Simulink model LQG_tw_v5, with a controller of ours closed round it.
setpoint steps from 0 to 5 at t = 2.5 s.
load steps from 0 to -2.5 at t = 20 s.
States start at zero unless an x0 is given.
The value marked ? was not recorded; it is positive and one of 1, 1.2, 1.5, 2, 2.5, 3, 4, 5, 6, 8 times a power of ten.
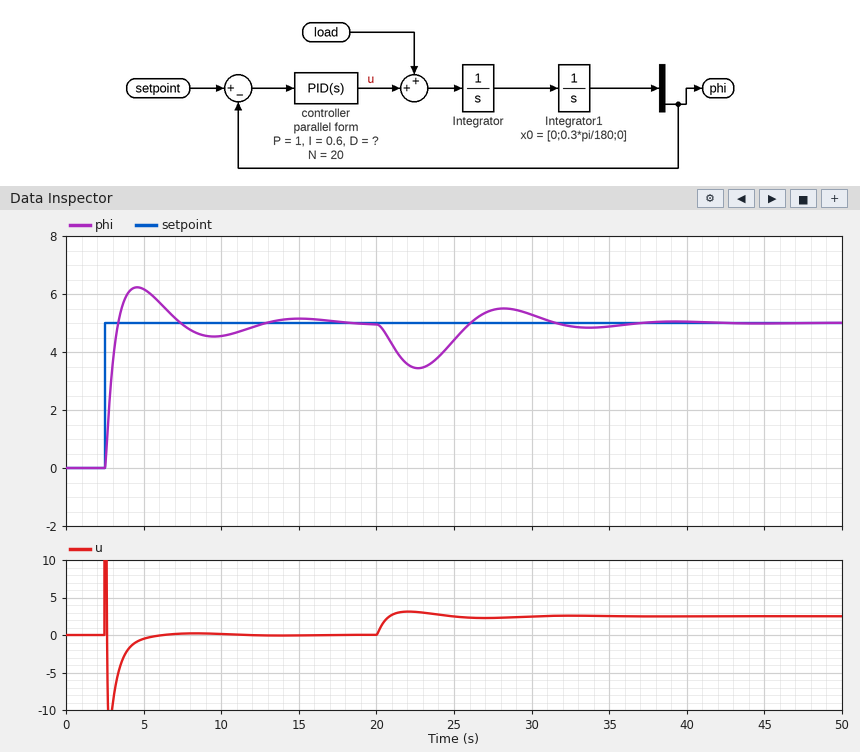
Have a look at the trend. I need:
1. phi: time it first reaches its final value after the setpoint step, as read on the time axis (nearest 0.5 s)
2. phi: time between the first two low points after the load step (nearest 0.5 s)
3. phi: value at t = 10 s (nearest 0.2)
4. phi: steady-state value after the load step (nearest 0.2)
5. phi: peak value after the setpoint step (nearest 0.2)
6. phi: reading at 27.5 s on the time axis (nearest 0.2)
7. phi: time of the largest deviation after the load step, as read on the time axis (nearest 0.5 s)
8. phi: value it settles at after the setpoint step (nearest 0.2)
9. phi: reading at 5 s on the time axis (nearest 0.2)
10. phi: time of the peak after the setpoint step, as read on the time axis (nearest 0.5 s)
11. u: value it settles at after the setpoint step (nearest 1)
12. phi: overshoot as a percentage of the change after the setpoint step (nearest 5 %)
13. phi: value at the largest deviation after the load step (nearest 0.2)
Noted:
3.5 s
11.0 s
4.6
5.0
6.2
5.4
22.5 s
5.0
6.2
4.5 s
0
25 %
3.4
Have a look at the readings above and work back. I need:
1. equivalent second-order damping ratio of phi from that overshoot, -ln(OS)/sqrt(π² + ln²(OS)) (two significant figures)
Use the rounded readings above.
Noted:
0.40
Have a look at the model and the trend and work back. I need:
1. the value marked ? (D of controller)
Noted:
2
